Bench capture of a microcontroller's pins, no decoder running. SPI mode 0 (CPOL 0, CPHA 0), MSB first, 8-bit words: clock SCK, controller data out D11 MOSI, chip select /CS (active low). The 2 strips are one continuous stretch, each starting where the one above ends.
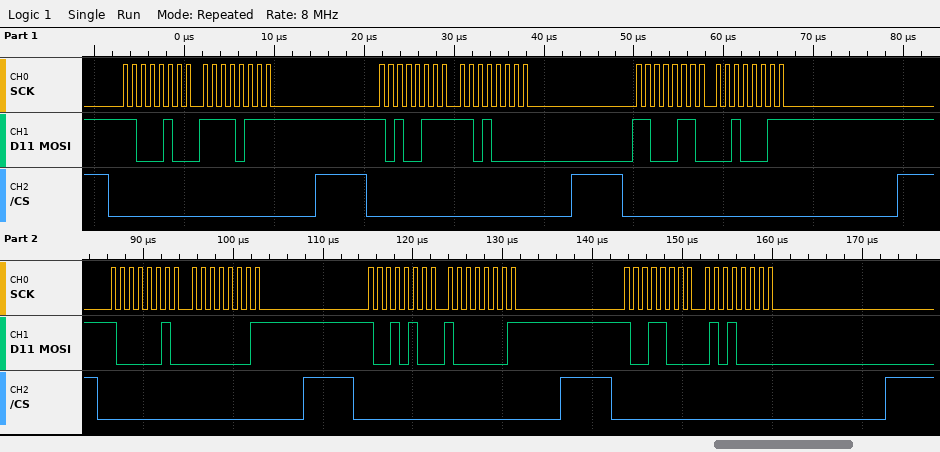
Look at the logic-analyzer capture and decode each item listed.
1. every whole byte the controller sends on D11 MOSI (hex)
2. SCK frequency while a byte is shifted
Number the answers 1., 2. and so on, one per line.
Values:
1. C4 F7 A7 D0 C6 23 82 01 94 81 98 50
2. 1 MHz
